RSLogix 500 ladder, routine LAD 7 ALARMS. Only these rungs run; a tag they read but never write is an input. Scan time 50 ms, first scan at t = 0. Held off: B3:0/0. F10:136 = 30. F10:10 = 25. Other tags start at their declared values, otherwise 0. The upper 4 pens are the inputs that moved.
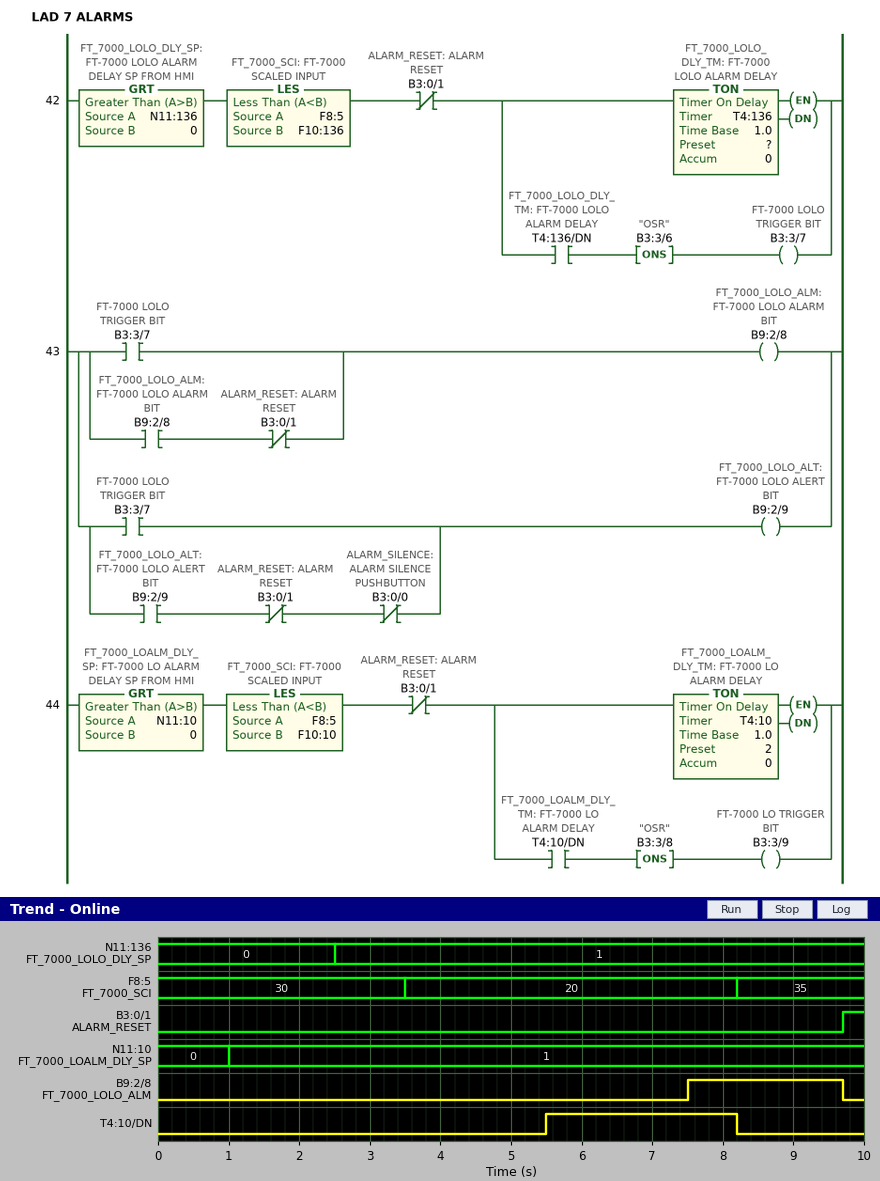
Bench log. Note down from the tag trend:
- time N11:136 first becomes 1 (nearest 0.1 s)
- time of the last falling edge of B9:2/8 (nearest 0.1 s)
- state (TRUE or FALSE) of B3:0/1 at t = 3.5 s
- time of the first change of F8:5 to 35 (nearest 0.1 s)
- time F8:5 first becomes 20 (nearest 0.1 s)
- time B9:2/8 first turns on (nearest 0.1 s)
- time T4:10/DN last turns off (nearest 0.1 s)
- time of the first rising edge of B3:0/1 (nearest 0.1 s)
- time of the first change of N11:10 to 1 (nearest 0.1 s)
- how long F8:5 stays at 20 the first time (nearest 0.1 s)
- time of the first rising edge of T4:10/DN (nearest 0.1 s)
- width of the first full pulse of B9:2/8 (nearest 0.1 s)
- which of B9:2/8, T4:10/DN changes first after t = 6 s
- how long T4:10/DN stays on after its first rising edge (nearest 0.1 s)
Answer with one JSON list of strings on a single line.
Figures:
["2.5 s", "9.7 s", "FALSE", "8.2 s", "3.5 s", "7.5 s", "8.2 s", "9.7 s", "1.0 s", "4.7 s", "5.5 s", "2.2 s", "B9:2/8", "2.7 s"]
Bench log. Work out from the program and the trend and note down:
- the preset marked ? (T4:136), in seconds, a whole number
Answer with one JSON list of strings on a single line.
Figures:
["4 s"]
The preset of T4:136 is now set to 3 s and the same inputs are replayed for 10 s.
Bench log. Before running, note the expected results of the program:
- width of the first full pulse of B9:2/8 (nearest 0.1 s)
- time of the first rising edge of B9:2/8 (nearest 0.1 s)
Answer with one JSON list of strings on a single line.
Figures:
["3.2 s", "6.5 s"]
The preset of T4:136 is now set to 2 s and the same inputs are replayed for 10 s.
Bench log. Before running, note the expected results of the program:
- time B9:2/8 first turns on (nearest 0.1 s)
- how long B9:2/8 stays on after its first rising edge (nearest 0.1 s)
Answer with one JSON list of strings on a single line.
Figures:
["5.5 s", "4.2 s"]
